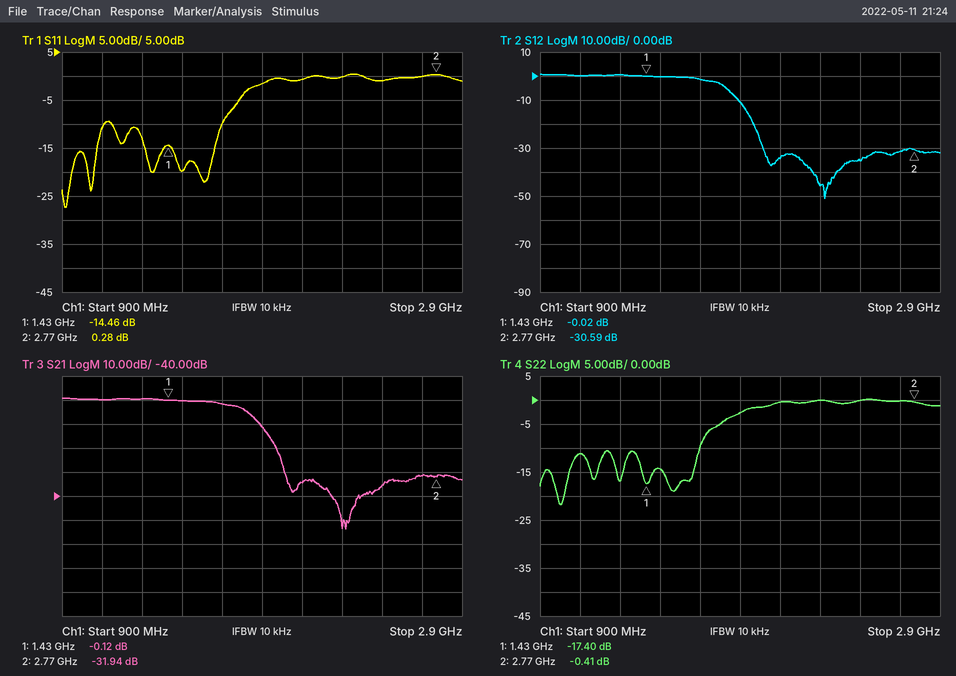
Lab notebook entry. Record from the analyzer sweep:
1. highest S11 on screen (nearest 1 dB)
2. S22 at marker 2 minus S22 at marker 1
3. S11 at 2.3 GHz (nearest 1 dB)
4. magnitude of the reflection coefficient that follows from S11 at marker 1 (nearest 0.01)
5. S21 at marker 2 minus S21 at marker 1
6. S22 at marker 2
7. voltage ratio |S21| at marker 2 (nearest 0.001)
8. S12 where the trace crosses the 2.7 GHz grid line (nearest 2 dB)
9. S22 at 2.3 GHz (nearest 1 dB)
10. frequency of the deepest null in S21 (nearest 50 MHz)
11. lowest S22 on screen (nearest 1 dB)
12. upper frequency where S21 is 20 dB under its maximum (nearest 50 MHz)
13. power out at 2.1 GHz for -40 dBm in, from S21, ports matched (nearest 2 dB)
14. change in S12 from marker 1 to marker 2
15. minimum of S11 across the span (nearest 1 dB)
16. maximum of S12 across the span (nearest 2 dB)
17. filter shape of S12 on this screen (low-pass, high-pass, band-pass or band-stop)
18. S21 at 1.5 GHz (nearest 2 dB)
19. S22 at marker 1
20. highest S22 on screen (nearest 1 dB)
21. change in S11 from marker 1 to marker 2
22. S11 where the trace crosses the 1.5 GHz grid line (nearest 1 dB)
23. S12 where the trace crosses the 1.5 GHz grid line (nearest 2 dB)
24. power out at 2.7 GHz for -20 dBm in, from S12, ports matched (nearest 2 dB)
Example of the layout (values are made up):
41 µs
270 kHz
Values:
0 dB
16.99 dB
0 dB
0.19
-31.82 dB
-0.41 dB
0.025
-32 dB
0 dB
2.30 GHz
-22 dB
1.95 GHz
-74 dBm
-30.57 dB
-27 dB
0 dB
low-pass
0 dB
-17.40 dB
0 dB
14.74 dB
-20 dB
0 dB
-52 dBm
